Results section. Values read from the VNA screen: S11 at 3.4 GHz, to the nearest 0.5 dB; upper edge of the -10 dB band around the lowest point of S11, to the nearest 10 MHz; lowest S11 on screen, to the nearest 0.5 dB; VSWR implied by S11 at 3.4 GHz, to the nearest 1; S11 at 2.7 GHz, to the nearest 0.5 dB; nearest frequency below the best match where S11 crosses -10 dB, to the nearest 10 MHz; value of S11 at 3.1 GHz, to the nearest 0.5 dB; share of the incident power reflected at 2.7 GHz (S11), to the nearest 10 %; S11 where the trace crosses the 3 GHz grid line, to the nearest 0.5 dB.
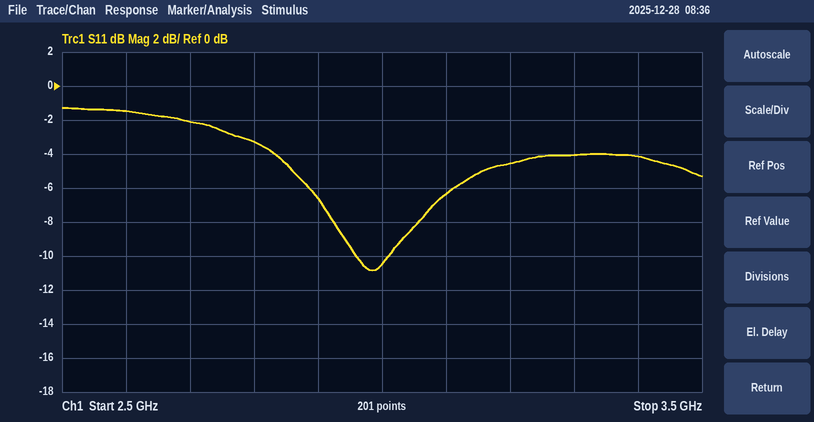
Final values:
-4.0 dB
3.01 GHz
-11.0 dB
4
-2.0 dB
2.96 GHz
-6.5 dB
60 %
-10.5 dB
